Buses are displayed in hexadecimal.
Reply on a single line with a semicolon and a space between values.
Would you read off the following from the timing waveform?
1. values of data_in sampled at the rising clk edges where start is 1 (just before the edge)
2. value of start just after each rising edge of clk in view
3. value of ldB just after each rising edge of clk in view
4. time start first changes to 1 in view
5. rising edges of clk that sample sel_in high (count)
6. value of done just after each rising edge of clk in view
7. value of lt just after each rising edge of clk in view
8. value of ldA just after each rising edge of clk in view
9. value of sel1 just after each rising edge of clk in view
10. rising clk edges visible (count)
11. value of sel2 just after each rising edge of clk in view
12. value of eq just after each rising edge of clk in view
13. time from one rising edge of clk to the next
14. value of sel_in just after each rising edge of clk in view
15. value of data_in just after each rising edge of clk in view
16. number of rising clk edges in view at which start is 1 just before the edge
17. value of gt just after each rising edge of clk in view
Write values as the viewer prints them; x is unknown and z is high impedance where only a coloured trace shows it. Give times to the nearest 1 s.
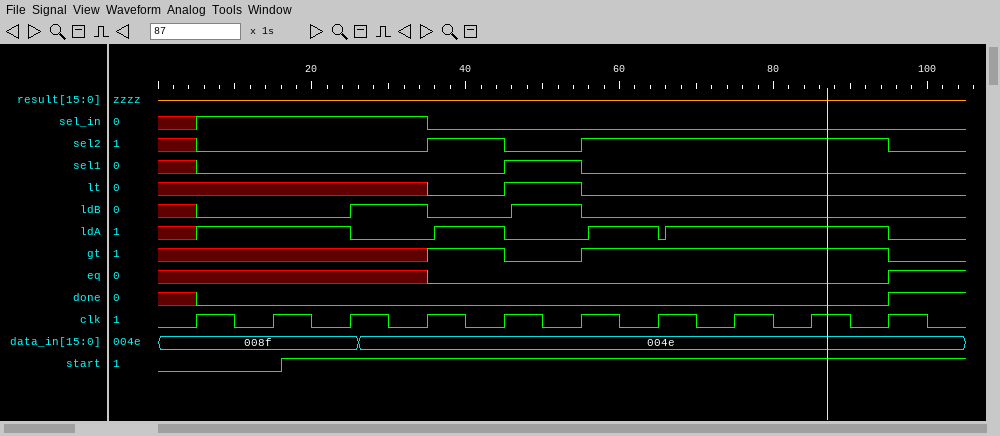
008f, 004e, 004e, 004e, 004e, 004e, 004e, 004e; 0 0 1 1 1 1 1 1 1 1; 0 0 1 0 0 0 0 0 0 0; 16 s; 3; 0 0 0 0 0 0 0 0 0 1; x x x 0 1 0 0 0 0 0; 1 1 0 0 0 0 0 1 1 0; 0 0 0 0 1 0 0 0 0 0; 10; 0 0 0 1 0 1 1 1 1 0; x x x 0 0 0 0 0 0 1; 10 s; 1 1 1 0 0 0 0 0 0 0; 008f, 008f, 008f, 004e, 004e, 004e, 004e, 004e, 004e, 004e; 8; x x x 1 0 1 1 1 1 0
